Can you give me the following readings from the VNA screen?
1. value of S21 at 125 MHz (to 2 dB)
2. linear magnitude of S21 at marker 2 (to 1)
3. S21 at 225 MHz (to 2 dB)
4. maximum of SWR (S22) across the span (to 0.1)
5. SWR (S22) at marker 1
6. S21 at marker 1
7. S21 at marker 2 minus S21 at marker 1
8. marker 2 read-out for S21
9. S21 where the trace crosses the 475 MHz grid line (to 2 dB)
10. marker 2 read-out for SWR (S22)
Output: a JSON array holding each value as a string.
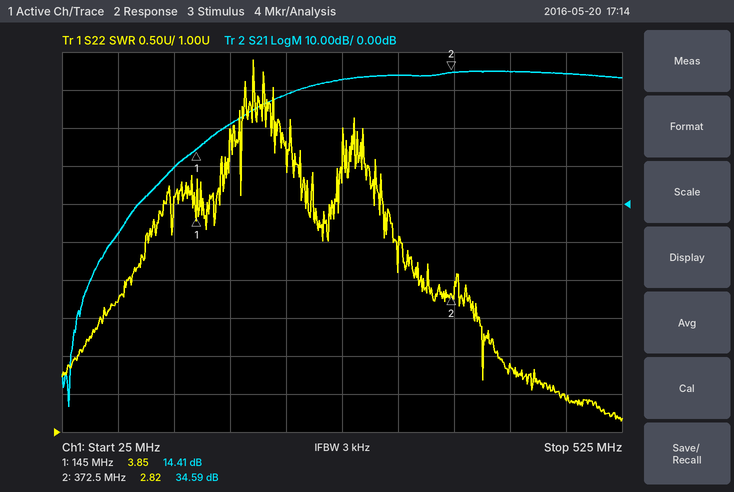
["10 dB", "54", "28 dB", "5.9", "3.85", "14.41 dB", "20.18 dB", "34.59 dB", "34 dB", "2.82"]
